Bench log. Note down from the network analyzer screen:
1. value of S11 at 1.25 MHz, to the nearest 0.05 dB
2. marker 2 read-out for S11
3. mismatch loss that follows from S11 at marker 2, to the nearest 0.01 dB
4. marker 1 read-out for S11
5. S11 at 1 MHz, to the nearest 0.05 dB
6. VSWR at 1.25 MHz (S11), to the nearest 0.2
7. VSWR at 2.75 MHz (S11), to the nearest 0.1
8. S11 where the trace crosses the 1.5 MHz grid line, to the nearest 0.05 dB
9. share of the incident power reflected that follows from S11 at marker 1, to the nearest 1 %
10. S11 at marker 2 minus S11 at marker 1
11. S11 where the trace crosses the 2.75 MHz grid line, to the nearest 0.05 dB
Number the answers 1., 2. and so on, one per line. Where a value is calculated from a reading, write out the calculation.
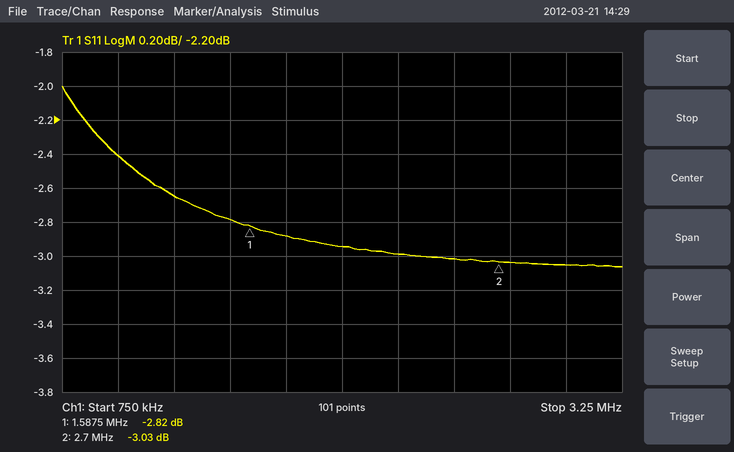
1. -2.65 dB
2. -3.03 dB
3. −10 log10(1 − 10^(-3.03/10)) ≈ 2.99 dB
4. -2.82 dB
5. -2.40 dB
6. |Γ| = 10^(-2.65/20) = 0.7371; VSWR = (1 + 0.7371)/(1 − 0.7371) ≈ 6.6
7. |Γ| = 10^(-3.05/20) = 0.7039; VSWR = (1 + 0.7039)/(1 − 0.7039) ≈ 5.8
8. -2.80 dB
9. 10^(-2.82/10) ≈ 52 %
10. -3.03 − (-2.82) = -0.21 dB
11. -3.05 dB
